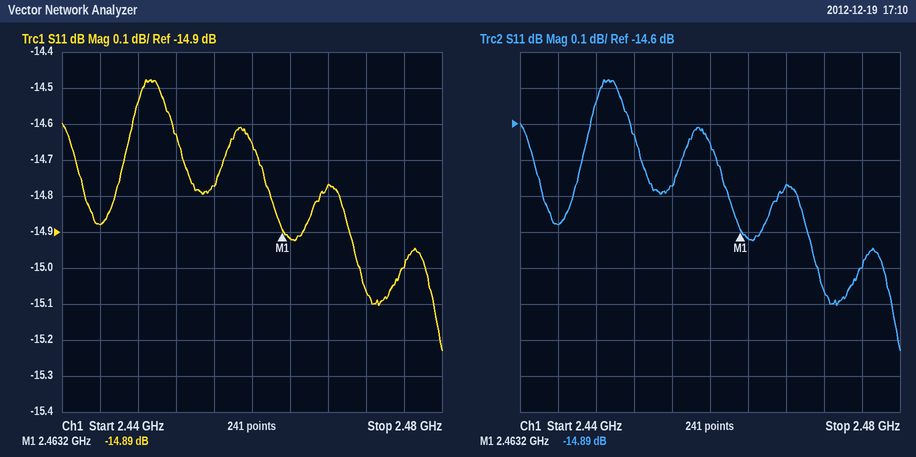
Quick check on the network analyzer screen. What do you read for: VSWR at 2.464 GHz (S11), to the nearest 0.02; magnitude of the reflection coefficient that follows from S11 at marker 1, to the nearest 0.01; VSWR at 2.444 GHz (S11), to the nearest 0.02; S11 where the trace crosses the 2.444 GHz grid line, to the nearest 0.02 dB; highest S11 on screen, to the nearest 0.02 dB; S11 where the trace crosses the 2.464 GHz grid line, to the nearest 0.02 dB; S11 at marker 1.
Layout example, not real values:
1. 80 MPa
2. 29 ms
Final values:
1. 1.44
2. 0.18
3. 1.44
4. -14.88 dB
5. -14.48 dB
6. -14.92 dB
7. -14.89 dB
